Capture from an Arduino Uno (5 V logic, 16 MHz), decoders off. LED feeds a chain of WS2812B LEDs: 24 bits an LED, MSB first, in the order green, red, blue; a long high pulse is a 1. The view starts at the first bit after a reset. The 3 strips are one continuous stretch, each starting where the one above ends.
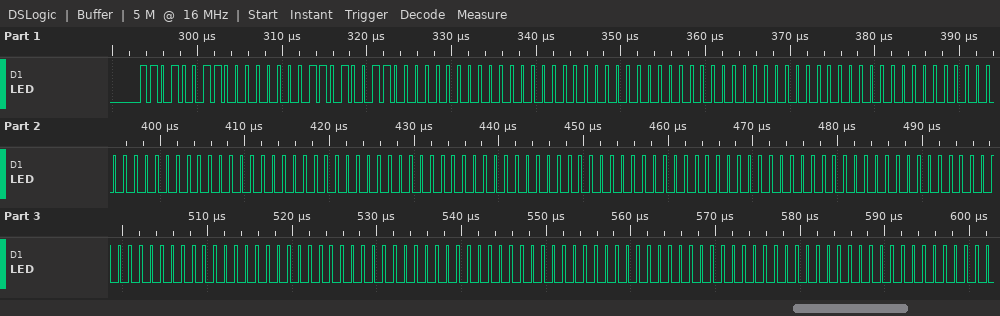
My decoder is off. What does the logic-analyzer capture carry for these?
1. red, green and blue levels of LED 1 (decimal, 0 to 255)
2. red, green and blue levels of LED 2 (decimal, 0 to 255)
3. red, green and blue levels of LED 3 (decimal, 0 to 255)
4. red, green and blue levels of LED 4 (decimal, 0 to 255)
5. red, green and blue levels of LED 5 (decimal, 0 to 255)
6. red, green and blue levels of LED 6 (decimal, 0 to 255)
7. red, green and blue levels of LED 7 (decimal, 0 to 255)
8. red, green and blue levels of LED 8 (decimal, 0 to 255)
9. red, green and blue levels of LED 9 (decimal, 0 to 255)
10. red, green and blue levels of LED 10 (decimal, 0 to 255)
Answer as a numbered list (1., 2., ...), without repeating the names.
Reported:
1. 0, 211, 211
2. 0, 0, 0
3. 0, 0, 0
4. 0, 0, 0
5. 0, 0, 0
6. 0, 0, 0
7. 0, 0, 0
8. 0, 0, 0
9. 0, 0, 0
10. 0, 0, 0
